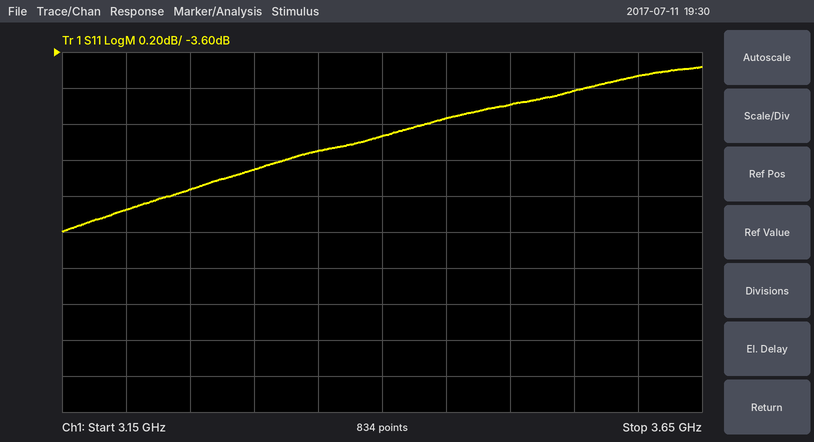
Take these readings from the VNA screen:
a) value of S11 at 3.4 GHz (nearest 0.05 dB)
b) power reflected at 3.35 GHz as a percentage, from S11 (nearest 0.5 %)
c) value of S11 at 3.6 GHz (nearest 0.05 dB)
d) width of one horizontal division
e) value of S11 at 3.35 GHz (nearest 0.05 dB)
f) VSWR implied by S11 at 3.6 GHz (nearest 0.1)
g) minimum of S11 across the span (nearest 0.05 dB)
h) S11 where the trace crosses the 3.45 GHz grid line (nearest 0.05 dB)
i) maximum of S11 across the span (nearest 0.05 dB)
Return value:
-4.05 dB
38.5 %
-3.75 dB
50 MHz
-4.15 dB
4.7
-4.60 dB
-3.95 dB
-3.70 dB
